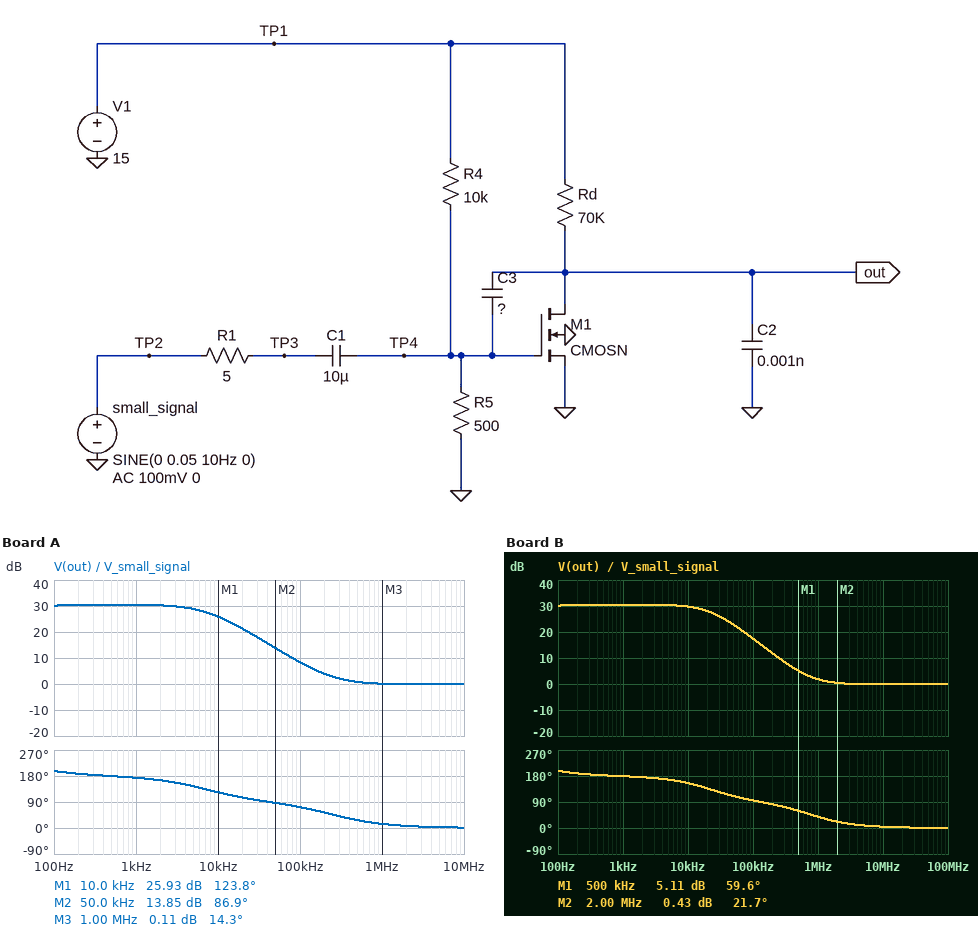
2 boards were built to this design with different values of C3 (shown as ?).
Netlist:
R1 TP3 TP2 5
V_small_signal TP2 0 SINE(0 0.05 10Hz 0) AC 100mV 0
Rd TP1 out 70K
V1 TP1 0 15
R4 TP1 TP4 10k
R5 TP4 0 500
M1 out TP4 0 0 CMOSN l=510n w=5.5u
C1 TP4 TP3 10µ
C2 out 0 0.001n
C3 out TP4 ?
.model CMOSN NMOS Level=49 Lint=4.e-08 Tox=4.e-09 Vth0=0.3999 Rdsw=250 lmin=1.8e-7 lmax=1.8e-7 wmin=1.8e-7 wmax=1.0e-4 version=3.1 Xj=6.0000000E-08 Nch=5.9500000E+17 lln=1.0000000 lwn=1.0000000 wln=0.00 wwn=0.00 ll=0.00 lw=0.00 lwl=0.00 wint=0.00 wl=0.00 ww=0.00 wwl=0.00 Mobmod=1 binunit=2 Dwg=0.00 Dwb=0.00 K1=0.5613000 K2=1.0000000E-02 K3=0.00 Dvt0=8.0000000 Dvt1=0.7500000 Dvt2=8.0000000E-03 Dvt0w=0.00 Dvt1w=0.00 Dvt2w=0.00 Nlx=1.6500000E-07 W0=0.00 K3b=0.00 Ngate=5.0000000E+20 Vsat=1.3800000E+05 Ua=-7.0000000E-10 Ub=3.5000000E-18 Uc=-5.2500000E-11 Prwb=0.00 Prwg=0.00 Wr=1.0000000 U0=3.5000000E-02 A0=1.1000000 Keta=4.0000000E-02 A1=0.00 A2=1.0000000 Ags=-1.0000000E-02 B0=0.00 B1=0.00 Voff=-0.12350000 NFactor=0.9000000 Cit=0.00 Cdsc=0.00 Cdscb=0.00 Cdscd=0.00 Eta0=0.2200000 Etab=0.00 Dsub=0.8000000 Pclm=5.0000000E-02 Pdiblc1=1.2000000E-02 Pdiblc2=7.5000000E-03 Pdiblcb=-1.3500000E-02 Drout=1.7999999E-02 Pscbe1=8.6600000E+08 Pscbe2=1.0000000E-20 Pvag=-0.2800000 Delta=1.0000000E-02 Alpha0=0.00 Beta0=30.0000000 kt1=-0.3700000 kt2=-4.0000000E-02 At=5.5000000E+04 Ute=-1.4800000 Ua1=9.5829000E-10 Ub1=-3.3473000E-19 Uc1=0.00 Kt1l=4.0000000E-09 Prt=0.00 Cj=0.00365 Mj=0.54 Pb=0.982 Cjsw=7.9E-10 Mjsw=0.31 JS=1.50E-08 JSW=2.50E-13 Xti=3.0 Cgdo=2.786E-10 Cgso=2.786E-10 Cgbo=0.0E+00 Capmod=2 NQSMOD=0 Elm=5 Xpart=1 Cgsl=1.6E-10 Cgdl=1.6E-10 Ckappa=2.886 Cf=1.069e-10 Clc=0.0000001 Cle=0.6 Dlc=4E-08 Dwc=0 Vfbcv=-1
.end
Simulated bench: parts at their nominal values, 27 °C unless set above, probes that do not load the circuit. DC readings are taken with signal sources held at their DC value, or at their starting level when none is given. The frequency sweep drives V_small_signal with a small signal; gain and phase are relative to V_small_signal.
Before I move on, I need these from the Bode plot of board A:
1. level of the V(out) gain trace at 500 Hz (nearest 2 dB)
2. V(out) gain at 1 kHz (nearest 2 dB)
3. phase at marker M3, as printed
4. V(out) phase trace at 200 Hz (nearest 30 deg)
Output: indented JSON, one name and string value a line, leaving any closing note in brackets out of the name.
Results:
{
  "level of the V(out) gain trace at 500 Hz": "30 dB",
  "V(out) gain at 1 kHz": "30 dB",
  "phase at marker M3, as printed": "14.3 deg",
  "V(out) phase trace at 200 Hz": "180 deg"
}
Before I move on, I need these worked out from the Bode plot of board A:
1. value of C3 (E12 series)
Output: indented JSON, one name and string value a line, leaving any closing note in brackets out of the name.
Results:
{
  "value of C3": "560 pF"
}
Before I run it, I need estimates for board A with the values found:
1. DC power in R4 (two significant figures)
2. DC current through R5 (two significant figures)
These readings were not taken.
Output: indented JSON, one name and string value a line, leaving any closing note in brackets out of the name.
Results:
{
  "DC power in R4": "20 mW",
  "DC current through R5": "1.4 mA"
}
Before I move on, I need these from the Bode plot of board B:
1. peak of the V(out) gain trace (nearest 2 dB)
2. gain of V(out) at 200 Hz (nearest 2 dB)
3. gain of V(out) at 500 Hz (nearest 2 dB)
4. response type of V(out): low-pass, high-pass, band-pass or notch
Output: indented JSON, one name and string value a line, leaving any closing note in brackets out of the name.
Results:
{
  "peak of the V(out) gain trace": "30 dB",
  "gain of V(out) at 200 Hz": "30 dB",
  "gain of V(out) at 500 Hz": "30 dB",
  "response type of V(out): low-pass, high-pass, band-pass or notch": "low-pass"
}
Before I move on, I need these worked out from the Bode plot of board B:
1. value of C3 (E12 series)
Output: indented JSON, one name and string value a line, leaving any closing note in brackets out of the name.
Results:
{
  "value of C3": "180 pF"
}
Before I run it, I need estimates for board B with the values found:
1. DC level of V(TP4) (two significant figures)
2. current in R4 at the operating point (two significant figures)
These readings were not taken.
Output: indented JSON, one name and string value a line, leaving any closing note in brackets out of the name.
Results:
{
  "DC level of V(TP4)": "710 mV",
  "current in R4 at the operating point": "1.4 mA"
}
